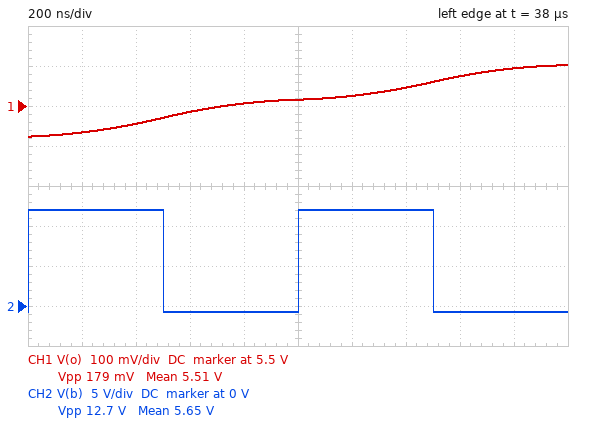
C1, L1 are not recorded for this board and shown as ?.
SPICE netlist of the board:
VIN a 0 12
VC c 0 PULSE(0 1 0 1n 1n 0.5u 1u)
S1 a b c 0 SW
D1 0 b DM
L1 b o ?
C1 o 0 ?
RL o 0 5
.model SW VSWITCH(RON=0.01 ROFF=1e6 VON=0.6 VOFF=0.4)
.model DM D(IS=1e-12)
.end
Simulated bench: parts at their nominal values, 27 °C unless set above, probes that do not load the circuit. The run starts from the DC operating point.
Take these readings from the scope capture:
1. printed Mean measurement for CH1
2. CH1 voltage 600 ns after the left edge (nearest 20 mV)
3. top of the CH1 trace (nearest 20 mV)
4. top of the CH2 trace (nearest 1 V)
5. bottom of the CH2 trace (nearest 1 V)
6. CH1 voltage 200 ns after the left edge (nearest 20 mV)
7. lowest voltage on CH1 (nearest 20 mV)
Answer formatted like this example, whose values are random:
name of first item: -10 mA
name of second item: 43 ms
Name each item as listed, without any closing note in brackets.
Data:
printed Mean measurement for CH1: 5.51 V
CH1 voltage 600 ns after the left edge: 5.48 V
top of the CH1 trace: 5.60 V
top of the CH2 trace: 12 V
bottom of the CH2 trace: -1 V
CH1 voltage 200 ns after the left edge: 5.44 V
lowest voltage on CH1: 5.42 V
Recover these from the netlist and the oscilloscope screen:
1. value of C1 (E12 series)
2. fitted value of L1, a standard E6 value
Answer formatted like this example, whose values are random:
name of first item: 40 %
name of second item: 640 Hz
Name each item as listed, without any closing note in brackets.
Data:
value of C1: 1.5 µF
fitted value of L1, a standard E6 value: 15 µH
